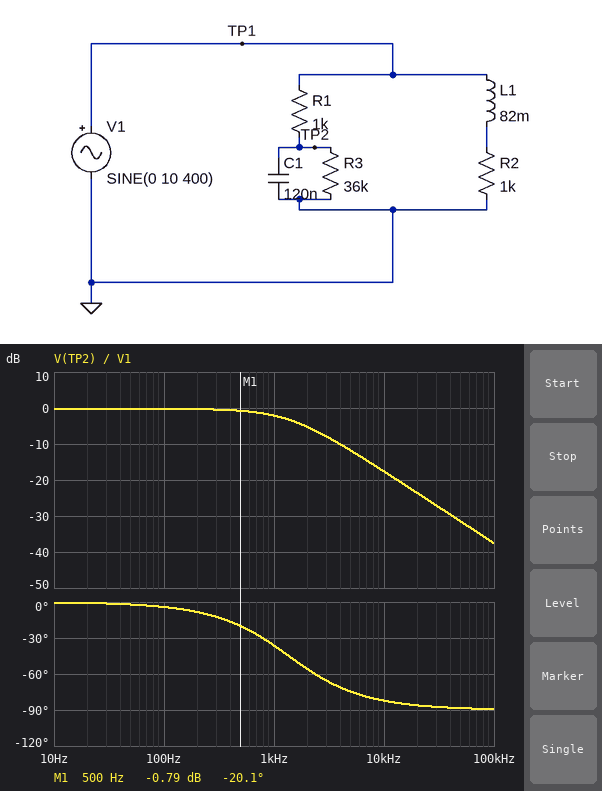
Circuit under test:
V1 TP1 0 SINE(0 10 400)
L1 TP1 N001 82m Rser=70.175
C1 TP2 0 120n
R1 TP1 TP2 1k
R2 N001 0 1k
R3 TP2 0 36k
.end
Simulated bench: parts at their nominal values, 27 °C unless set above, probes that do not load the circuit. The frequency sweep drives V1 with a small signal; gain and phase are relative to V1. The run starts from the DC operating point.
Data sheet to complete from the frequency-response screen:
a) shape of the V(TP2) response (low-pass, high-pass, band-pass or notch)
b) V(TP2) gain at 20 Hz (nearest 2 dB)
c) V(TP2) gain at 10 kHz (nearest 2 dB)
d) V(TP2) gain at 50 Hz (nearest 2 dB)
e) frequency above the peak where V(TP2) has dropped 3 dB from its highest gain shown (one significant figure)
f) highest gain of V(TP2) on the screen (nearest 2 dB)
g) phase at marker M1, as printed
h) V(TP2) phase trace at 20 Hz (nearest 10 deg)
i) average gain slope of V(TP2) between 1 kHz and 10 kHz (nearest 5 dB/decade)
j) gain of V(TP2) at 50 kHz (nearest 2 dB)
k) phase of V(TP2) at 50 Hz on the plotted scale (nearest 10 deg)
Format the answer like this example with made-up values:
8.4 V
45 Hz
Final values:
low-pass
0 dB
-18 dB
0 dB
1 kHz
0 dB
-20.1 deg
0 deg
-15 dB/decade
-32 dB
0 deg
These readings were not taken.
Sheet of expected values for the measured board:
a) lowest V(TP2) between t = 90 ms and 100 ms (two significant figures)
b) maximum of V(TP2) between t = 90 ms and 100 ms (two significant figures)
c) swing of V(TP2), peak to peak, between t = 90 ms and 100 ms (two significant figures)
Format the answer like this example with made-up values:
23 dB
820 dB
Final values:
-9.3 V
9.3 V
19 V
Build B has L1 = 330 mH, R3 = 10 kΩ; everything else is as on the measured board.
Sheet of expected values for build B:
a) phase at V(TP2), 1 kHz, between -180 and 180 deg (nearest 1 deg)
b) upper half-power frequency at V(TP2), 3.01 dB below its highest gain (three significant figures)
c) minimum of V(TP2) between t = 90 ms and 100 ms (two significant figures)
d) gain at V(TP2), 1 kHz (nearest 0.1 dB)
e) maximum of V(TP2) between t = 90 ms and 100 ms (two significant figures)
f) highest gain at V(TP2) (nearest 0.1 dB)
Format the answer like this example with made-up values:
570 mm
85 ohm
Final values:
-34 deg
1.46 kHz
-8.8 V
-2.5 dB
8.8 V
-0.8 dB
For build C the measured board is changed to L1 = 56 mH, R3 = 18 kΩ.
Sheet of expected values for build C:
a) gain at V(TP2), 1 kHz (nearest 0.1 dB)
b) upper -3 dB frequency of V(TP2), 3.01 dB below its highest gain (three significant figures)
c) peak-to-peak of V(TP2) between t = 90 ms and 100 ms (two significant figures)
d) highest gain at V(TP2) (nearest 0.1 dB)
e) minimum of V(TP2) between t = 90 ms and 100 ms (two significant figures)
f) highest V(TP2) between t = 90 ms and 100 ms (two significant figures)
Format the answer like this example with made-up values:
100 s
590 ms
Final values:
-2.3 dB
1.40 kHz
18 V
-0.5 dB
-9.1 V
9.1 V
